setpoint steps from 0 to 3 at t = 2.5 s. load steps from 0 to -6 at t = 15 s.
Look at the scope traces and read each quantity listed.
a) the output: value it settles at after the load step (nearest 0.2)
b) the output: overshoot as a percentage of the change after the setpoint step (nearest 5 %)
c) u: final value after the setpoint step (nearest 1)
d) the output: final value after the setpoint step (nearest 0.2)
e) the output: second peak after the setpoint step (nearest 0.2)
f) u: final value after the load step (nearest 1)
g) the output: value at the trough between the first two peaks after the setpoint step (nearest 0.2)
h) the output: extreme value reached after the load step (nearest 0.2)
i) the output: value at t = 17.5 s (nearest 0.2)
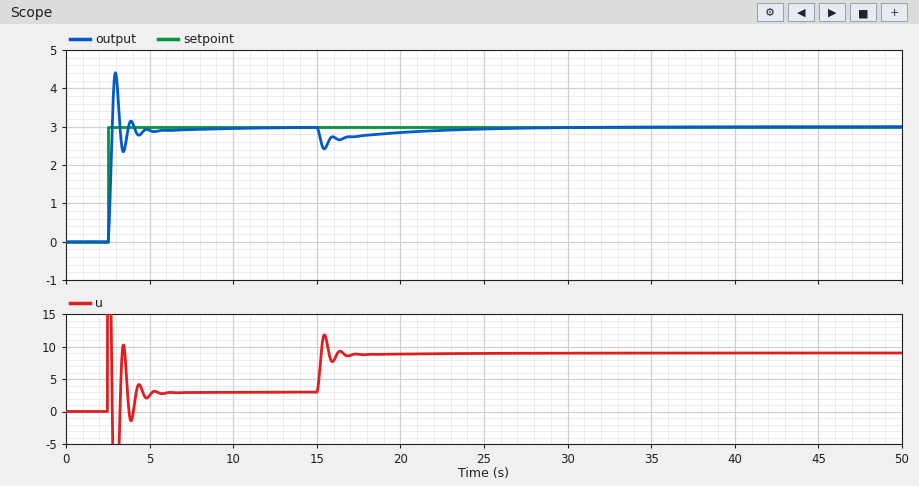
3.0
45 %
3
3.0
3.2
9
2.4
2.4
2.8
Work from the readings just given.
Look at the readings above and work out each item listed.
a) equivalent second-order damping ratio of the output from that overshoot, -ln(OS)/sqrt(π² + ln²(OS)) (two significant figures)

0.25
